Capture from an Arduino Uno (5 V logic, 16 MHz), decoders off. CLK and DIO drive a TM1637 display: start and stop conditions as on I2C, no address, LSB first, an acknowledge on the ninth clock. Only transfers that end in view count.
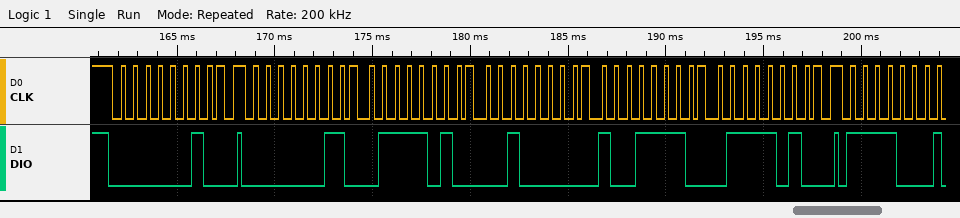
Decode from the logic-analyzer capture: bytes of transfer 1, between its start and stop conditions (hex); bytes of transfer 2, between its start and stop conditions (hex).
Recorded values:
40
C0 5E 04 79 5E
